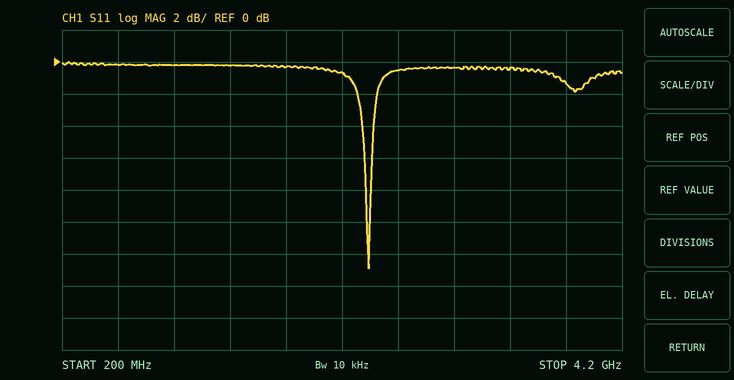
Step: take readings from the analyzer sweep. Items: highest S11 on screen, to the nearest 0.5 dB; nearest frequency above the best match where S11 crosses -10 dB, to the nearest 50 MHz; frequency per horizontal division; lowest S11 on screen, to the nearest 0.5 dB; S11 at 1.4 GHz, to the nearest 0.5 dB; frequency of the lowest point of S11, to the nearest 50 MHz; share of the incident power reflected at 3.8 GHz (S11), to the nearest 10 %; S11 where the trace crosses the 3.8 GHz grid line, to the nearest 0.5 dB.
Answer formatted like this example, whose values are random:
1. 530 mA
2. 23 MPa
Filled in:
1. 0.0 dB
2. 2.40 GHz
3. 400 MHz
4. -13.0 dB
5. 0.0 dB
6. 2.40 GHz
7. 70 %
8. -1.5 dB
